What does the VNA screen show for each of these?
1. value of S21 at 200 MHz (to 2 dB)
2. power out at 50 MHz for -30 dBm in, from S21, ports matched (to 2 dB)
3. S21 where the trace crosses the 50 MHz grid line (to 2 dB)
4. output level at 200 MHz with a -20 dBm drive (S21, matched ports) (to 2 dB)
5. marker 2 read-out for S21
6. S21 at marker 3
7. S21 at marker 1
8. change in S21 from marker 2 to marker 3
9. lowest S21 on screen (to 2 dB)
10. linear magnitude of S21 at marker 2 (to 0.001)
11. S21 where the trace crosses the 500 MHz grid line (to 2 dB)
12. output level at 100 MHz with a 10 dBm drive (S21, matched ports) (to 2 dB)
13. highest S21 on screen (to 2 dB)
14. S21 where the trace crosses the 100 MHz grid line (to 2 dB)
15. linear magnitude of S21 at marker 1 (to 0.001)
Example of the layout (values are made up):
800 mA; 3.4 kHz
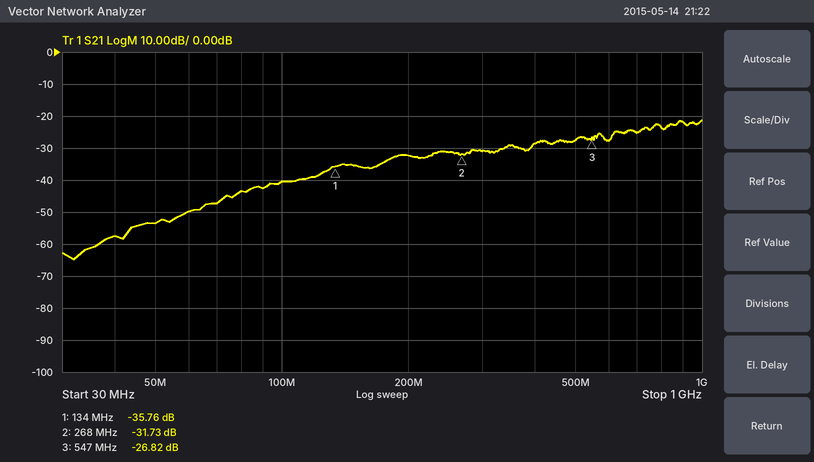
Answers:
-32 dB; -84 dBm; -54 dB; -52 dBm; -31.73 dB; -26.82 dB; -35.76 dB; 4.91 dB; -64 dB; 0.026; -28 dB; -30 dBm; -22 dB; -40 dB; 0.016
